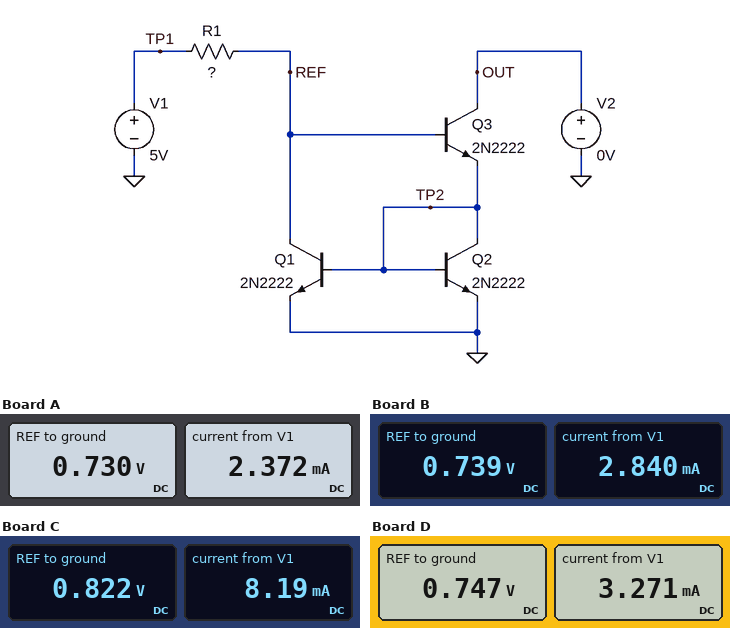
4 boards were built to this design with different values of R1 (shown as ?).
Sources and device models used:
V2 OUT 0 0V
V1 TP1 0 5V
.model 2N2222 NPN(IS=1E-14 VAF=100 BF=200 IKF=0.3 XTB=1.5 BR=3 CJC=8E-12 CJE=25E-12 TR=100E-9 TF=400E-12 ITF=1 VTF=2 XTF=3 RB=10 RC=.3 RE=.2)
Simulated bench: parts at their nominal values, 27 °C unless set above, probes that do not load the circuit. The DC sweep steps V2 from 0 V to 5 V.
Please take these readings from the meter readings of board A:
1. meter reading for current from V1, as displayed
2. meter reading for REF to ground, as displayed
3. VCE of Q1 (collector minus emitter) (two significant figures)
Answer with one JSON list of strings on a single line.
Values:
["2.372 mA", "0.730 V", "730 mV"]
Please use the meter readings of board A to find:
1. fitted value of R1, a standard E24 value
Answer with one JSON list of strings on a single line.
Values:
["1.8 kΩ"]
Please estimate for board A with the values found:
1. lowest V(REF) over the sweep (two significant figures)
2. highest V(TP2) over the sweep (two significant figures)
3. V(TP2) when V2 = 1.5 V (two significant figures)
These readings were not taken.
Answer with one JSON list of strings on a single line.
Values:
["730 mV", "670 mV", "670 mV"]
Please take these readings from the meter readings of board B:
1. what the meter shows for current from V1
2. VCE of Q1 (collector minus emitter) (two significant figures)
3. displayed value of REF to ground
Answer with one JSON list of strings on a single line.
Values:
["2.840 mA", "740 mV", "0.739 V"]
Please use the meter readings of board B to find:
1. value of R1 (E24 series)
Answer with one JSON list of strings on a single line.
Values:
["1.5 kΩ"]
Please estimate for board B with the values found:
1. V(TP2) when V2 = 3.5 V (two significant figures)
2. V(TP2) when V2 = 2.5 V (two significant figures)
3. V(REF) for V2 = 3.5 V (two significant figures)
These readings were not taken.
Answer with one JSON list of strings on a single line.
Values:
["680 mV", "680 mV", "1.4 V"]
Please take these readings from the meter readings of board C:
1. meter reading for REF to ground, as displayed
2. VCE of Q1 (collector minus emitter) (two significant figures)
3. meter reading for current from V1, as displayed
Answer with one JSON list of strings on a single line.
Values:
["0.822 V", "820 mV", "8.19 mA"]
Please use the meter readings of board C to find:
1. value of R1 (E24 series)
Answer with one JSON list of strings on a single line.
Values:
["510 Ω"]
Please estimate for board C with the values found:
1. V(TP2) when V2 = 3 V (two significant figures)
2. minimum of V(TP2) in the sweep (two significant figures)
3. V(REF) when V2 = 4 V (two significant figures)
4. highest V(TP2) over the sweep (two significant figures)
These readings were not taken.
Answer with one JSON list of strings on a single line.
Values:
["710 mV", "2.6 mV", "1.4 V", "710 mV"]
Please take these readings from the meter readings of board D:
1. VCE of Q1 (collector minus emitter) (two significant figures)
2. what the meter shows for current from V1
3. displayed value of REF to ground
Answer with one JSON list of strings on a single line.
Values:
["750 mV", "3.271 mA", "0.747 V"]
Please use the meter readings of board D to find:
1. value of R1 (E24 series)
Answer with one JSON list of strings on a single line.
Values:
["1.3 kΩ"]
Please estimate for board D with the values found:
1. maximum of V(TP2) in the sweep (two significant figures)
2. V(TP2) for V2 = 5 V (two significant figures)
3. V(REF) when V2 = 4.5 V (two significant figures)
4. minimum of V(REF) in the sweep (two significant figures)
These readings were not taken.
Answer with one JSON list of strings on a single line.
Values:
["680 mV", "680 mV", "1.4 V", "750 mV"]
